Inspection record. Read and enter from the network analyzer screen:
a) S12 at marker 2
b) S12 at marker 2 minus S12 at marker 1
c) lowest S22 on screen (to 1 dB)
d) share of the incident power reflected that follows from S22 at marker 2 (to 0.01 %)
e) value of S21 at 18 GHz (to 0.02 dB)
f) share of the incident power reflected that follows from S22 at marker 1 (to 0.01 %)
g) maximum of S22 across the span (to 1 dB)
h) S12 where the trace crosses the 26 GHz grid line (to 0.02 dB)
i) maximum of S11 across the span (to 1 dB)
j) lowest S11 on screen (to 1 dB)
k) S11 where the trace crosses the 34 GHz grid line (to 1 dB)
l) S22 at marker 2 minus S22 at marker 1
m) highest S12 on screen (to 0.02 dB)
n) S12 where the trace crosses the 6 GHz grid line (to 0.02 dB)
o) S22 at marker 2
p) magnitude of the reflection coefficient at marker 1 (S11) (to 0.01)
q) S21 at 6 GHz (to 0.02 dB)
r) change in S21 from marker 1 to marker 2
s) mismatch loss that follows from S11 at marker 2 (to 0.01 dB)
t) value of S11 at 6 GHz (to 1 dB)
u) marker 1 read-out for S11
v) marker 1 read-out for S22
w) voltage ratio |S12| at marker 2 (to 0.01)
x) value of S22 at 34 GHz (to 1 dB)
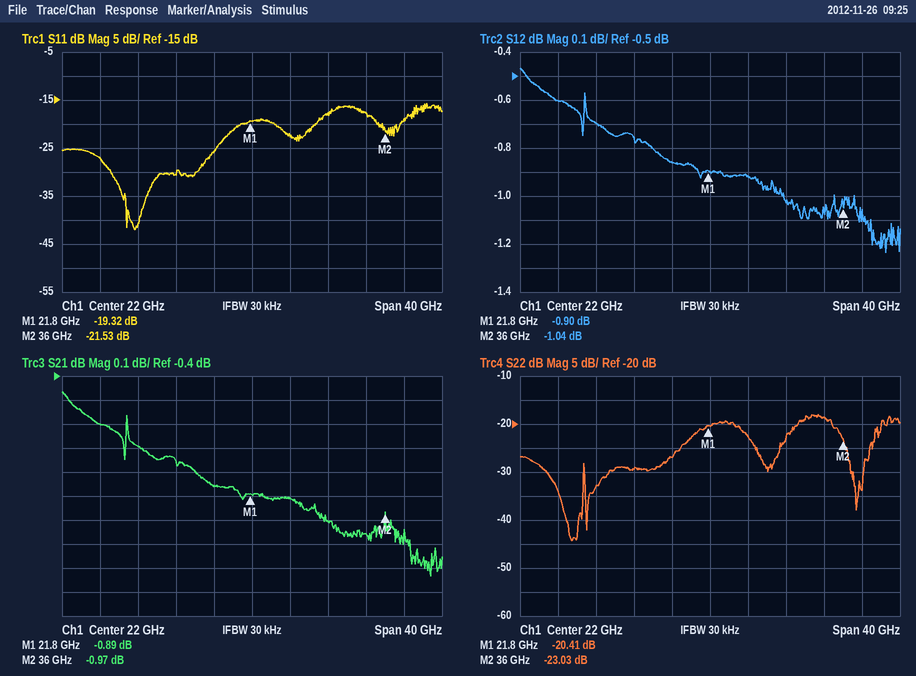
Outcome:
-1.04 dB
-0.14 dB
-44 dB
0.50 %
-0.86 dB
0.91 %
-18 dB
-0.92 dB
-16 dB
-42 dB
-18 dB
-2.62 dB
-0.46 dB
-0.60 dB
-23.03 dB
0.11
-0.60 dB
-0.08 dB
0.03 dB
-27 dB
-19.32 dB
-20.41 dB
0.89
-19 dB
